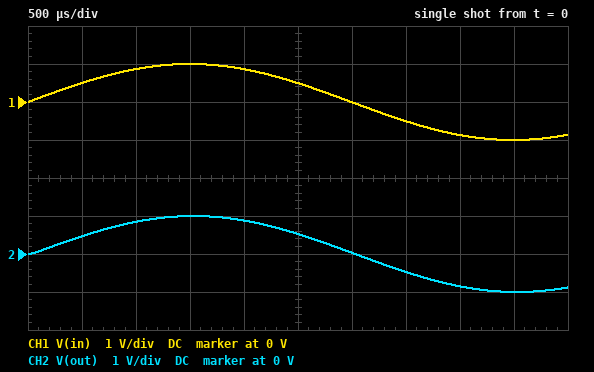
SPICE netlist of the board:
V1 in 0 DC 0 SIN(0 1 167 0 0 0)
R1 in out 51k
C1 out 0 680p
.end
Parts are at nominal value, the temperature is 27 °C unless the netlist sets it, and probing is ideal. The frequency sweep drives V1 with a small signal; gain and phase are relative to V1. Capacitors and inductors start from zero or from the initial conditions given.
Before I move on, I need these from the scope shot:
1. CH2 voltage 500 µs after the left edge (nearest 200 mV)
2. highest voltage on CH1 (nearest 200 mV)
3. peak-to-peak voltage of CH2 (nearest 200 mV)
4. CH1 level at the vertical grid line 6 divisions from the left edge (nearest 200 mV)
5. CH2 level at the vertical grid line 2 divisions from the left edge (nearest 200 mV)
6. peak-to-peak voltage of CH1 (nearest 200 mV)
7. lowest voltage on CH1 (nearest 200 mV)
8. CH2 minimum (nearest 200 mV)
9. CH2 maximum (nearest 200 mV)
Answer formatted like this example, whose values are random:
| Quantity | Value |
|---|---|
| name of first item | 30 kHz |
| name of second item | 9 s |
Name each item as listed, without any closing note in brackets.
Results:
| Quantity | Value |
|---|---|
| CH2 voltage 500 µs after the left edge | 400 mV |
| highest voltage on CH1 | 1.0 V |
| peak-to-peak voltage of CH2 | 2.0 V |
| CH1 level at the vertical grid line 6 divisions from the left edge | 0 V |
| CH2 level at the vertical grid line 2 divisions from the left edge | 800 mV |
| peak-to-peak voltage of CH1 | 2.0 V |
| lowest voltage on CH1 | -1.0 V |
| CH2 minimum | -1.0 V |
| CH2 maximum | 1.0 V |
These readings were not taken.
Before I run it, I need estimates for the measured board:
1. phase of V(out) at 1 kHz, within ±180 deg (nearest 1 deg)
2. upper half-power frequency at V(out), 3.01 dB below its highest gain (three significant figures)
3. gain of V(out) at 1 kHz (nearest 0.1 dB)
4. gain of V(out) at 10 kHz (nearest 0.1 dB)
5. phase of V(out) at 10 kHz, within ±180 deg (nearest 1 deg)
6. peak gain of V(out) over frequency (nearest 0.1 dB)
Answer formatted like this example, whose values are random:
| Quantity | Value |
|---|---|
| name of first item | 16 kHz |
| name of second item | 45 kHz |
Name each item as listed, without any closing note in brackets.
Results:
| Quantity | Value |
|---|---|
| phase of V(out) at 1 kHz, within ±180 deg | -12 deg |
| upper half-power frequency at V(out), 3.01 dB below its highest gain | 4.59 kHz |
| gain of V(out) at 1 kHz | -0.2 dB |
| gain of V(out) at 10 kHz | -7.6 dB |
| phase of V(out) at 10 kHz, within ±180 deg | -65 deg |
| peak gain of V(out) over frequency | 0 dB |
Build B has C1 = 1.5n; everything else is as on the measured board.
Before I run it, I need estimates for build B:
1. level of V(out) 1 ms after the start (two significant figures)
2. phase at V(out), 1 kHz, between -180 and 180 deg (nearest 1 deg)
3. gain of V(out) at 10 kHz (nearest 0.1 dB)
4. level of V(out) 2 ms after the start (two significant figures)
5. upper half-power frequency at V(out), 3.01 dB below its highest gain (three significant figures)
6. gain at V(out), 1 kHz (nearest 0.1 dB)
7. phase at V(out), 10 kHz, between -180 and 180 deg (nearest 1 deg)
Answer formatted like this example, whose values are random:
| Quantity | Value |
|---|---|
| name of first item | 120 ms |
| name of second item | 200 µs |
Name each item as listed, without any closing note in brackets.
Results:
| Quantity | Value |
|---|---|
| level of V(out) 1 ms after the start | 820 mV |
| phase at V(out), 1 kHz, between -180 and 180 deg | -26 deg |
| gain of V(out) at 10 kHz | -13.8 dB |
| level of V(out) 2 ms after the start | 900 mV |
| upper half-power frequency at V(out), 3.01 dB below its highest gain | 2.08 kHz |
| gain at V(out), 1 kHz | -0.9 dB |
| phase at V(out), 10 kHz, between -180 and 180 deg | -78 deg |
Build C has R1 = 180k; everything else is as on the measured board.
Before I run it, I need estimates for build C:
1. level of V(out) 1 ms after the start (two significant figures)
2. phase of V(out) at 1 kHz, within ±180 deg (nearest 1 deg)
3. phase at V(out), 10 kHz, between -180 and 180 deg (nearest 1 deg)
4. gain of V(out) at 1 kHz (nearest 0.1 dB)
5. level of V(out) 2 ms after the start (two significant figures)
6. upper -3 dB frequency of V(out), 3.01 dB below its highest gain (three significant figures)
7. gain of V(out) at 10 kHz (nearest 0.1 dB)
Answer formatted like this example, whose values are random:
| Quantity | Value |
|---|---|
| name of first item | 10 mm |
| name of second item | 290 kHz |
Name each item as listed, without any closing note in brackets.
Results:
| Quantity | Value |
|---|---|
| level of V(out) 1 ms after the start | 790 mV |
| phase of V(out) at 1 kHz, within ±180 deg | -38 deg |
| phase at V(out), 10 kHz, between -180 and 180 deg | -83 deg |
| gain of V(out) at 1 kHz | -2.0 dB |
| level of V(out) 2 ms after the start | 910 mV |
| upper -3 dB frequency of V(out), 3.01 dB below its highest gain | 1.30 kHz |
| gain of V(out) at 10 kHz | -17.8 dB |
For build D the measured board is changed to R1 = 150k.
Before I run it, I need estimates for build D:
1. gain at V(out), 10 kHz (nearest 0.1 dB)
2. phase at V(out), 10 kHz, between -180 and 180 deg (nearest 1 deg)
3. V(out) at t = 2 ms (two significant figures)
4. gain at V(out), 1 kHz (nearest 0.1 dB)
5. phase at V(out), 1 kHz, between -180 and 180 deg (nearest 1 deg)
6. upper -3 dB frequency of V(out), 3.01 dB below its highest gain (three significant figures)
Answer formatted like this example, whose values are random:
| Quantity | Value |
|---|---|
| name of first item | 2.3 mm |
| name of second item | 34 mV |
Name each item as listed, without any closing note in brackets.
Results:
| Quantity | Value |
|---|---|
| gain at V(out), 10 kHz | -16.2 dB |
| phase at V(out), 10 kHz, between -180 and 180 deg | -81 deg |
| V(out) at t = 2 ms | 910 mV |
| gain at V(out), 1 kHz | -1.5 dB |
| phase at V(out), 1 kHz, between -180 and 180 deg | -33 deg |
| upper -3 dB frequency of V(out), 3.01 dB below its highest gain | 1.56 kHz |
